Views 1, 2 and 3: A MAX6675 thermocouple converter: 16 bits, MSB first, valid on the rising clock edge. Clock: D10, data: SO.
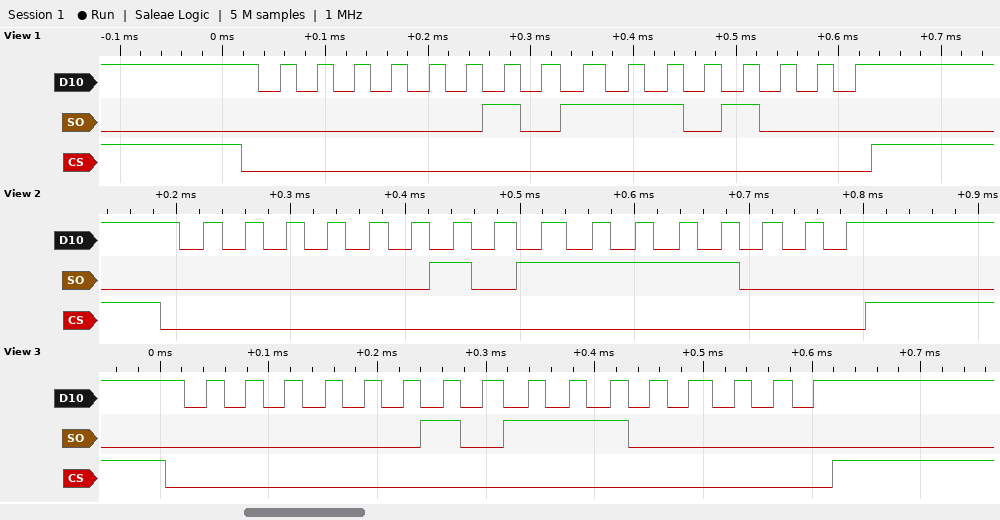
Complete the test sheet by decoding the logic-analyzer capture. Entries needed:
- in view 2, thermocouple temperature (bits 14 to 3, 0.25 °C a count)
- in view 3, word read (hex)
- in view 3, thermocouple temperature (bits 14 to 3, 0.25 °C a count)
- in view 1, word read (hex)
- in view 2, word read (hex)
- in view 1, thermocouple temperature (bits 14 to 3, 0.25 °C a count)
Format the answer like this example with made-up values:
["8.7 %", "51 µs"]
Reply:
["23.75 °C", "0x02E0", "23.00 °C", "0x02E8", "0x02F8", "23.25 °C"]
